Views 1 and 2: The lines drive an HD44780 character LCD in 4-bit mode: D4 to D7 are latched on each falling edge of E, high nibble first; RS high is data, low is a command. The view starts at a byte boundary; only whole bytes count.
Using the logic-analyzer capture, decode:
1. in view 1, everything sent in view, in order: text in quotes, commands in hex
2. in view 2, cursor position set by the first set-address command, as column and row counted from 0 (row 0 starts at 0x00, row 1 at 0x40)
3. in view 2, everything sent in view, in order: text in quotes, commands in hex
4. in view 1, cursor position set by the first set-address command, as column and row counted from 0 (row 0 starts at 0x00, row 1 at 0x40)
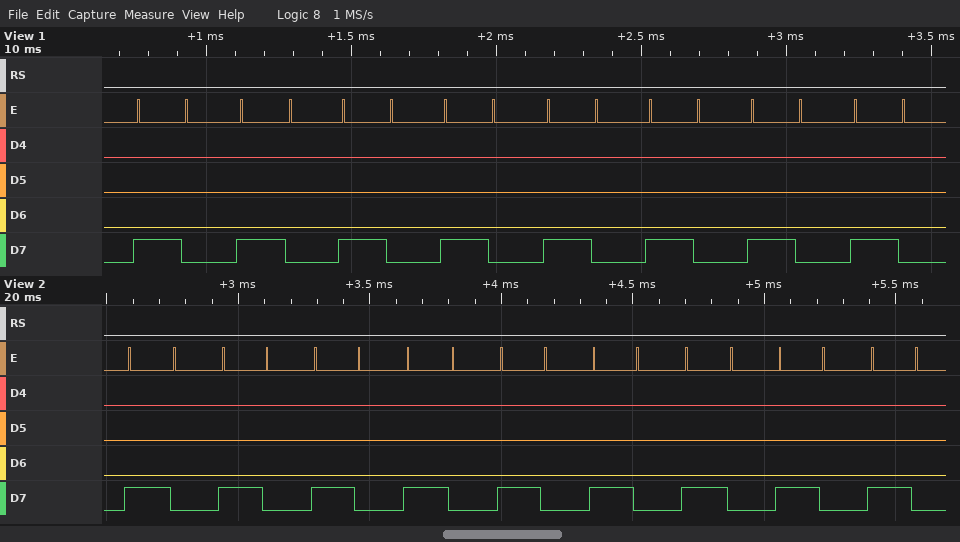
0x80 0x80 0x80 0x80 0x80 0x80 0x80 0x80
column 0, row 0
0x80 0x80 0x80 0x80 0x80 0x80 0x80 0x80 0x80
column 0, row 0
